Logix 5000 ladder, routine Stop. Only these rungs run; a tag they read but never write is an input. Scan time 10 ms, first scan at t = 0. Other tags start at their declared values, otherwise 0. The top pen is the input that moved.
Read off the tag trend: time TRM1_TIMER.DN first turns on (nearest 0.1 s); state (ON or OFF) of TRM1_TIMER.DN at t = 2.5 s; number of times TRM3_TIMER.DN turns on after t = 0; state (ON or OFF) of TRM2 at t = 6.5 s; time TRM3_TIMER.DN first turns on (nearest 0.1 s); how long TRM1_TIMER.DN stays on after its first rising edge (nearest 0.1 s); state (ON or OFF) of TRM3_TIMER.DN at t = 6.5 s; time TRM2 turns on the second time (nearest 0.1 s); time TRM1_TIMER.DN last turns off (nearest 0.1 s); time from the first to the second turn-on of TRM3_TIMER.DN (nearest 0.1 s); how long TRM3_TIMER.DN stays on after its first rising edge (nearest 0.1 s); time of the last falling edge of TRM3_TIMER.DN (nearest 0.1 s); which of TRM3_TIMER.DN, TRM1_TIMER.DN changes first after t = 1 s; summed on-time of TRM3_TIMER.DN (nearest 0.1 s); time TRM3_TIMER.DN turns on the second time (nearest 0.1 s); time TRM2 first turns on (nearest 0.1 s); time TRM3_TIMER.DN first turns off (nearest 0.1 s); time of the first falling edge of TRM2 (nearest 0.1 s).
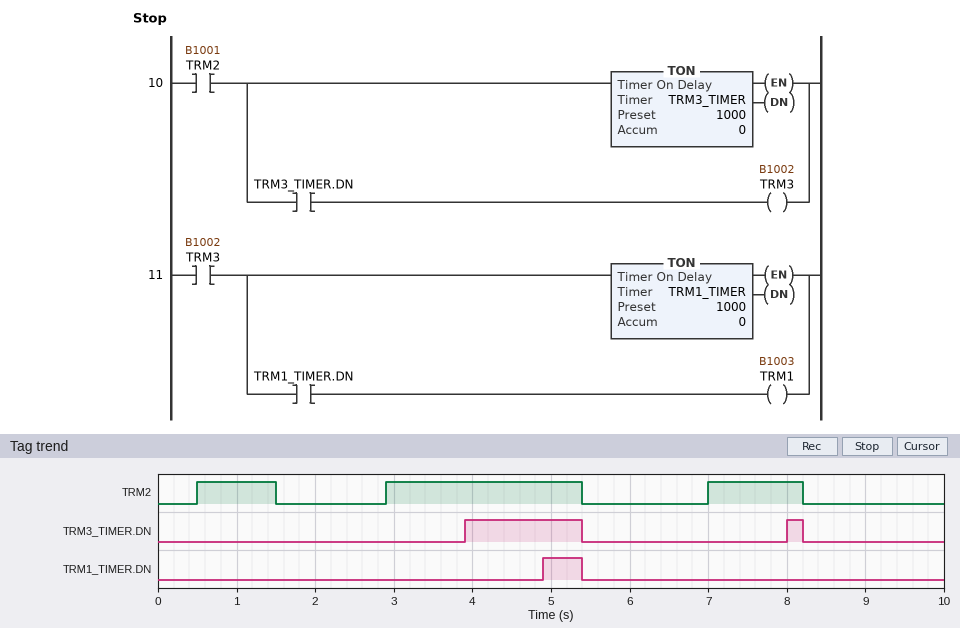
4.9 s
OFF
2
OFF
3.9 s
0.5 s
OFF
2.9 s
5.4 s
4.1 s
1.5 s
8.2 s
TRM3_TIMER.DN
1.7 s
8.0 s
0.5 s
5.4 s
1.5 s
